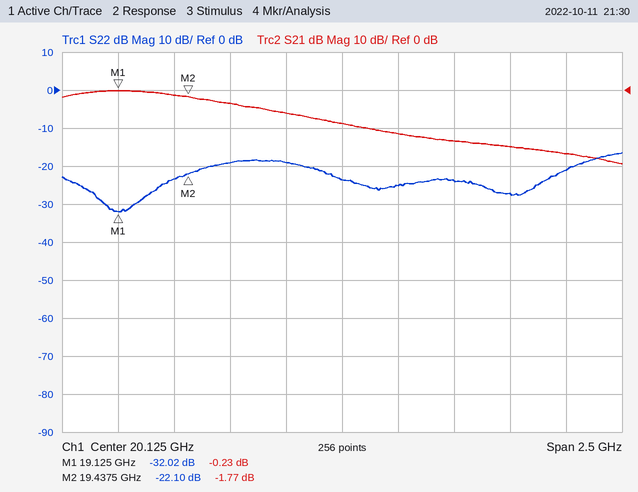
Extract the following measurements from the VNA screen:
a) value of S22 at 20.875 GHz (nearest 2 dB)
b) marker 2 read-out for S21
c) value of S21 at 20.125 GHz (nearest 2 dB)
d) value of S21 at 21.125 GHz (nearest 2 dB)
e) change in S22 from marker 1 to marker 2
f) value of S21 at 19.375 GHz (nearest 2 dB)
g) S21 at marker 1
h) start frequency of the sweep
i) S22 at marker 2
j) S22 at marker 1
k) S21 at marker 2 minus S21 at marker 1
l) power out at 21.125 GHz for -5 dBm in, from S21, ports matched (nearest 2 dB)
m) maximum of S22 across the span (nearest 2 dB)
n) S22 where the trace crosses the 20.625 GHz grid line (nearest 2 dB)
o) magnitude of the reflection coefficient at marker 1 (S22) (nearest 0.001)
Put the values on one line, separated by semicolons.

-28 dB; -1.77 dB; -8 dB; -16 dB; 9.92 dB; -2 dB; -0.23 dB; 18.875 GHz; -22.10 dB; -32.02 dB; -1.54 dB; -22 dBm; -16 dB; -24 dB; 0.025
